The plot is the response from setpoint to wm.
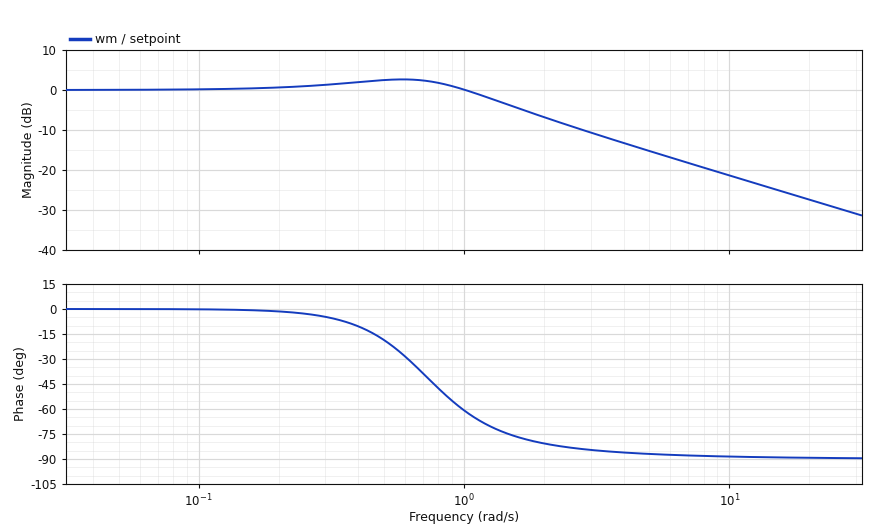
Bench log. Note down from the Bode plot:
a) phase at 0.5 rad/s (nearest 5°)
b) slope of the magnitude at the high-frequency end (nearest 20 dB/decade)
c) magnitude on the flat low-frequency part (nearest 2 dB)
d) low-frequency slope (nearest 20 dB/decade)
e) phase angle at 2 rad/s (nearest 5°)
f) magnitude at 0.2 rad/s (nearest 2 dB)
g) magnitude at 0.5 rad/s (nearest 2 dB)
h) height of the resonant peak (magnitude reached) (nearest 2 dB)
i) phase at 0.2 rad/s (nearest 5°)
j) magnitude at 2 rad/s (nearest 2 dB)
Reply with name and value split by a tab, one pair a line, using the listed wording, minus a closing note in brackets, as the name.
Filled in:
phase at 0.5 rad/s	-20°
slope of the magnitude at the high-frequency end	-20 dB/decade
magnitude on the flat low-frequency part	0 dB
low-frequency slope	0 dB/decade
phase angle at 2 rad/s	-80°
magnitude at 0.2 rad/s	0 dB
magnitude at 0.5 rad/s	2 dB
height of the resonant peak (magnitude reached)	2 dB
phase at 0.2 rad/s	0°
magnitude at 2 rad/s	-6 dB
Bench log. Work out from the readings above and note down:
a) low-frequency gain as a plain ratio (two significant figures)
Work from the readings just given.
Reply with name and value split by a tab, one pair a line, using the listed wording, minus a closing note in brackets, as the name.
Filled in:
low-frequency gain as a plain ratio	1.0
